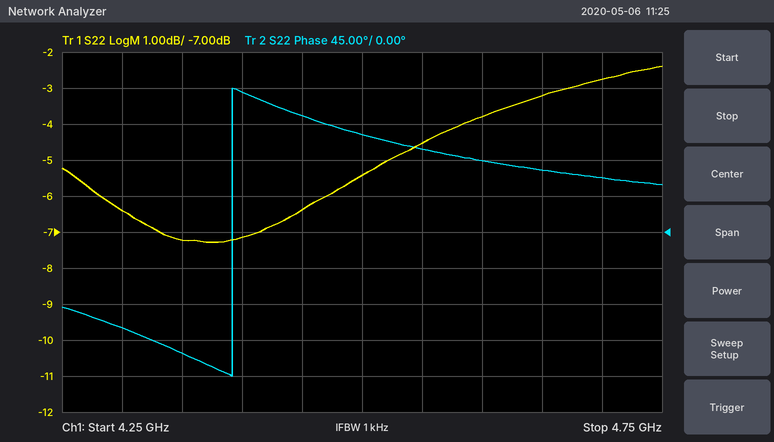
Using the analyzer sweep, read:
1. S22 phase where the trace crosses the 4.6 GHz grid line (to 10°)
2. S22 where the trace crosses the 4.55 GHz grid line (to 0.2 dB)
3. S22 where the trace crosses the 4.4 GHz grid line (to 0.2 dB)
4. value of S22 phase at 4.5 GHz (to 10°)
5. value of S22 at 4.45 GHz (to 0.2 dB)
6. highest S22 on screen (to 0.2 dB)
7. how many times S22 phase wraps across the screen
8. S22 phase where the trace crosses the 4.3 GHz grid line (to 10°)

90°
-4.6 dB
-7.2 dB
120°
-6.4 dB
-2.4 dB
1
-120°
